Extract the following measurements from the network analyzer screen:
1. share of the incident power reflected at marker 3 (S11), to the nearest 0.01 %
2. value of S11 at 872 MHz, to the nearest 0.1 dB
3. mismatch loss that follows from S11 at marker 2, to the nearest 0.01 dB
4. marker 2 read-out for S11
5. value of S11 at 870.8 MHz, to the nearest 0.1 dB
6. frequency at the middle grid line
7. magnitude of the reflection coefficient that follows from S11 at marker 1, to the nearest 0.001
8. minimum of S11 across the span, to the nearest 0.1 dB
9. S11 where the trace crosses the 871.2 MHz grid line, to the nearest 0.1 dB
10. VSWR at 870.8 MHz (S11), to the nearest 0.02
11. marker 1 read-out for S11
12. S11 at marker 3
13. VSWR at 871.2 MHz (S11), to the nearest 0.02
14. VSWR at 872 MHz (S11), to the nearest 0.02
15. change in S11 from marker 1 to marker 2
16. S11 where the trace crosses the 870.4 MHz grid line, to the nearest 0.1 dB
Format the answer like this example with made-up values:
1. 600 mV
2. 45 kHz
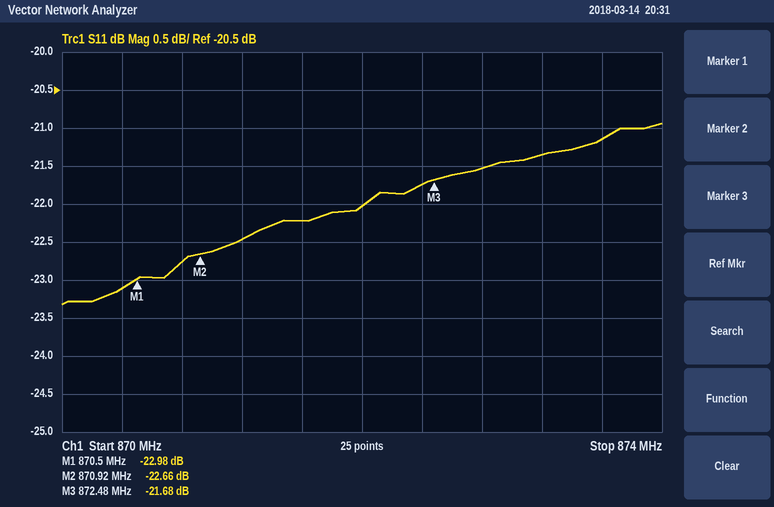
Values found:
1. 0.68 %
2. -22.0 dB
3. 0.02 dB
4. -22.66 dB
5. -22.8 dB
6. 872 MHz
7. 0.071
8. -23.3 dB
9. -22.5 dB
10. 1.16
11. -22.98 dB
12. -21.68 dB
13. 1.16
14. 1.18
15. 0.32 dB
16. -23.1 dB
